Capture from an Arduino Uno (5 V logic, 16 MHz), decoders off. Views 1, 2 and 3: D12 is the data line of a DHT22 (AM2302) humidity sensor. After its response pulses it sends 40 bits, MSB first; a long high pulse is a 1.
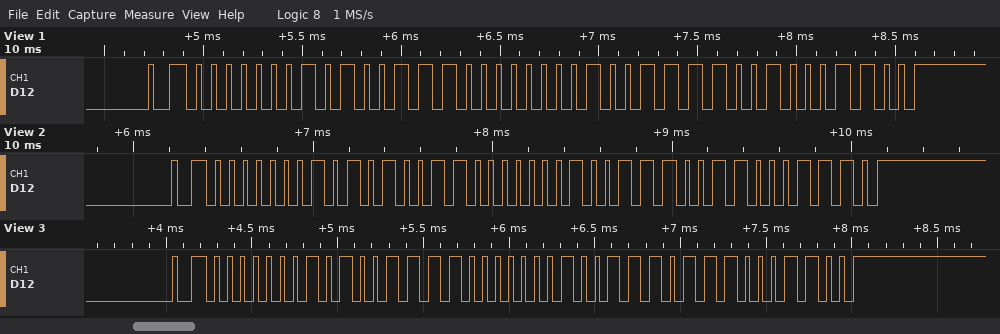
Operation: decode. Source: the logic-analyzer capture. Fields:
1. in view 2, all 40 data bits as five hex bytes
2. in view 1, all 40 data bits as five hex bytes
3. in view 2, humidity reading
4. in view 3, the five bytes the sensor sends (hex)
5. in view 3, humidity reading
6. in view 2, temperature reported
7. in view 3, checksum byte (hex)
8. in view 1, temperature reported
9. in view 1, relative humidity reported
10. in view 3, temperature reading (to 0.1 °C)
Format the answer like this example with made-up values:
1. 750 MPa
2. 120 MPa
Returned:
1. 01 53 01 39 8E
2. 01 4E 01 3C 8C
3. 33.9 %
4. 01 4F 01 3B 8C
5. 33.5 %
6. 31.3 °C
7. 0x8C
8. 31.6 °C
9. 33.4 %
10. 31.5 °C
